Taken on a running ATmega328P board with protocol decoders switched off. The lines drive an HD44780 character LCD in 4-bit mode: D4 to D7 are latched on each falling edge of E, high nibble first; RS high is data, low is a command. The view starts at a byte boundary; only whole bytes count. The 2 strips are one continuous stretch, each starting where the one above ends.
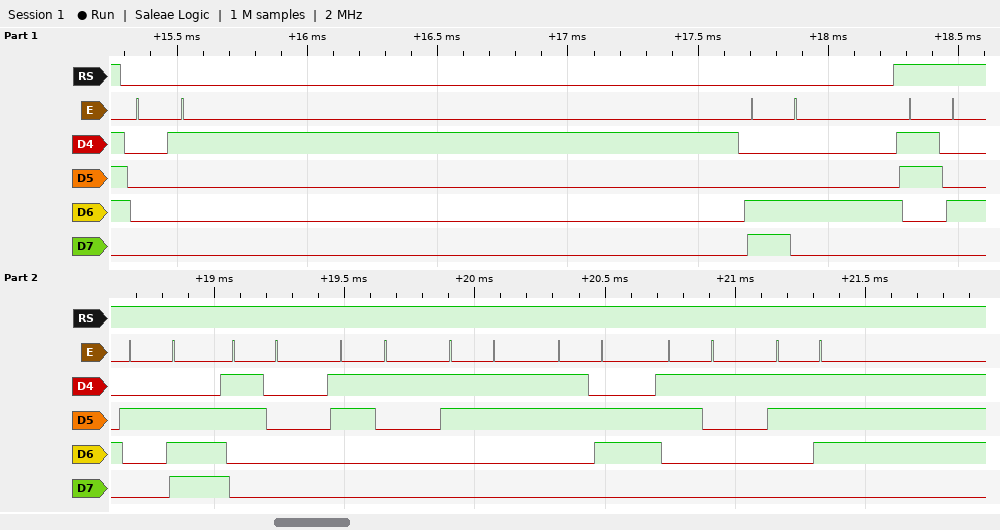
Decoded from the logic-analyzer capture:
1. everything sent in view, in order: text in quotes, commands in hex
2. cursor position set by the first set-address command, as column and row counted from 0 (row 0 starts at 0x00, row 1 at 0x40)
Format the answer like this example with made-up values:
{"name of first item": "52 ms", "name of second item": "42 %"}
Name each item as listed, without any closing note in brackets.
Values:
{"everything sent in view, in order: text in quotes, commands in hex": "0x01 0xC4 \"4.013617\"", "cursor position set by the first set-address command, as column and row counted from 0": "column 4, row 1"}
